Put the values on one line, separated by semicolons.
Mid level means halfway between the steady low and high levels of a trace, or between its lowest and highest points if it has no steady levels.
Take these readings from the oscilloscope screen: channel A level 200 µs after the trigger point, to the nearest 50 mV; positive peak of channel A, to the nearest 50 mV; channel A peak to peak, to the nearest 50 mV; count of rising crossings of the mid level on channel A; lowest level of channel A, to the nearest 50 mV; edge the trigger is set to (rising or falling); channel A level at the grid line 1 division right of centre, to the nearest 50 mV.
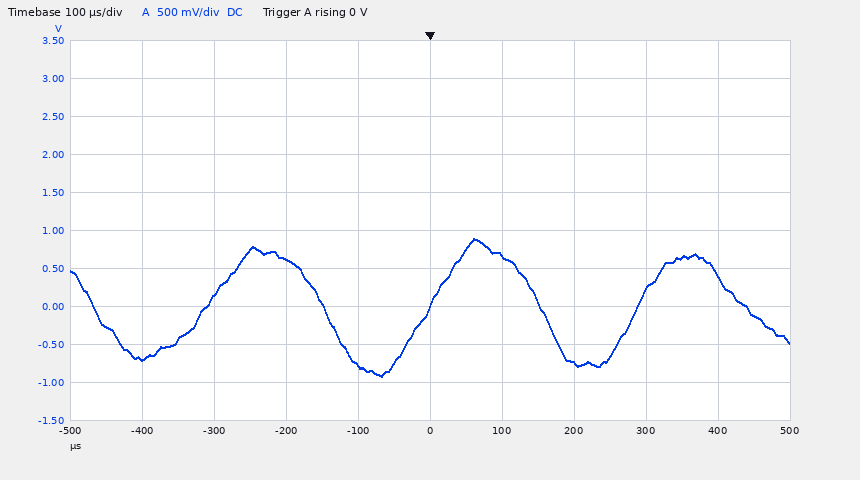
-750 mV; 900 mV; 1.80 V; 3; -900 mV; rising; 650 mV
